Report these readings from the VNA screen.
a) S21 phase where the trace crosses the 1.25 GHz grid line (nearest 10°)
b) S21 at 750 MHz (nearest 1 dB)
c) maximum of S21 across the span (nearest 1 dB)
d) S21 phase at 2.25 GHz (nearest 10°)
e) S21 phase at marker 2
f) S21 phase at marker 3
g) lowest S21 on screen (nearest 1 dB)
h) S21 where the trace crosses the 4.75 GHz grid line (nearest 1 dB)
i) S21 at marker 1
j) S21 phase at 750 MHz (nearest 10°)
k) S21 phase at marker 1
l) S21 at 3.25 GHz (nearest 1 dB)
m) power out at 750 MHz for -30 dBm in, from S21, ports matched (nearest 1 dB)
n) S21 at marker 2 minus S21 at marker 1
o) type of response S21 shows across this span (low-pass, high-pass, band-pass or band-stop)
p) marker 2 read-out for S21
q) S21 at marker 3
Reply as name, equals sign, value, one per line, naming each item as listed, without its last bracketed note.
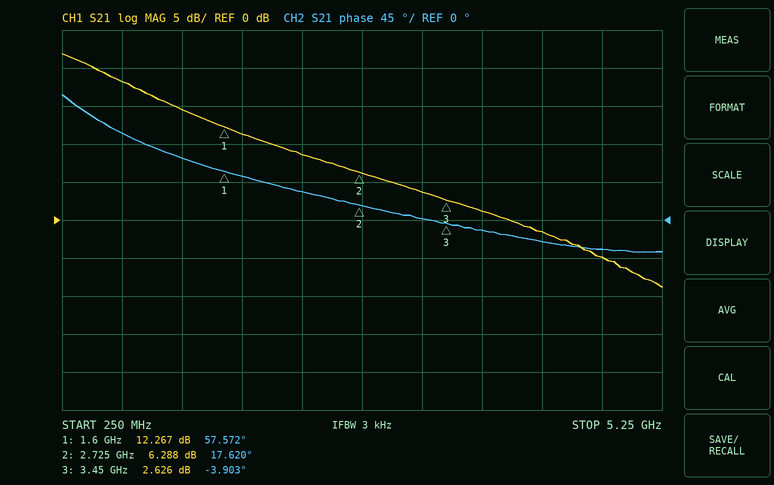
S21 phase where the trace crosses the 1.25 GHz grid line = 70°
S21 at 750 MHz = 18 dB
maximum of S21 across the span = 22 dB
S21 phase at 2.25 GHz = 30°
S21 phase at marker 2 = 17.620°
S21 phase at marker 3 = -3.903°
lowest S21 on screen = -9 dB
S21 where the trace crosses the 4.75 GHz grid line = -5 dB
S21 at marker 1 = 12.267 dB
S21 phase at 750 MHz = 100°
S21 phase at marker 1 = 57.572°
S21 at 3.25 GHz = 4 dB
power out at 750 MHz for -30 dBm in, from S21, ports matched = -12 dBm
S21 at marker 2 minus S21 at marker 1 = -5.979 dB
type of response S21 shows across this span = low-pass
marker 2 read-out for S21 = 6.288 dB
S21 at marker 3 = 2.626 dB
